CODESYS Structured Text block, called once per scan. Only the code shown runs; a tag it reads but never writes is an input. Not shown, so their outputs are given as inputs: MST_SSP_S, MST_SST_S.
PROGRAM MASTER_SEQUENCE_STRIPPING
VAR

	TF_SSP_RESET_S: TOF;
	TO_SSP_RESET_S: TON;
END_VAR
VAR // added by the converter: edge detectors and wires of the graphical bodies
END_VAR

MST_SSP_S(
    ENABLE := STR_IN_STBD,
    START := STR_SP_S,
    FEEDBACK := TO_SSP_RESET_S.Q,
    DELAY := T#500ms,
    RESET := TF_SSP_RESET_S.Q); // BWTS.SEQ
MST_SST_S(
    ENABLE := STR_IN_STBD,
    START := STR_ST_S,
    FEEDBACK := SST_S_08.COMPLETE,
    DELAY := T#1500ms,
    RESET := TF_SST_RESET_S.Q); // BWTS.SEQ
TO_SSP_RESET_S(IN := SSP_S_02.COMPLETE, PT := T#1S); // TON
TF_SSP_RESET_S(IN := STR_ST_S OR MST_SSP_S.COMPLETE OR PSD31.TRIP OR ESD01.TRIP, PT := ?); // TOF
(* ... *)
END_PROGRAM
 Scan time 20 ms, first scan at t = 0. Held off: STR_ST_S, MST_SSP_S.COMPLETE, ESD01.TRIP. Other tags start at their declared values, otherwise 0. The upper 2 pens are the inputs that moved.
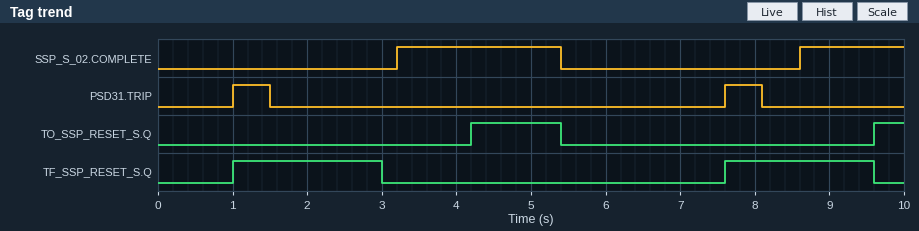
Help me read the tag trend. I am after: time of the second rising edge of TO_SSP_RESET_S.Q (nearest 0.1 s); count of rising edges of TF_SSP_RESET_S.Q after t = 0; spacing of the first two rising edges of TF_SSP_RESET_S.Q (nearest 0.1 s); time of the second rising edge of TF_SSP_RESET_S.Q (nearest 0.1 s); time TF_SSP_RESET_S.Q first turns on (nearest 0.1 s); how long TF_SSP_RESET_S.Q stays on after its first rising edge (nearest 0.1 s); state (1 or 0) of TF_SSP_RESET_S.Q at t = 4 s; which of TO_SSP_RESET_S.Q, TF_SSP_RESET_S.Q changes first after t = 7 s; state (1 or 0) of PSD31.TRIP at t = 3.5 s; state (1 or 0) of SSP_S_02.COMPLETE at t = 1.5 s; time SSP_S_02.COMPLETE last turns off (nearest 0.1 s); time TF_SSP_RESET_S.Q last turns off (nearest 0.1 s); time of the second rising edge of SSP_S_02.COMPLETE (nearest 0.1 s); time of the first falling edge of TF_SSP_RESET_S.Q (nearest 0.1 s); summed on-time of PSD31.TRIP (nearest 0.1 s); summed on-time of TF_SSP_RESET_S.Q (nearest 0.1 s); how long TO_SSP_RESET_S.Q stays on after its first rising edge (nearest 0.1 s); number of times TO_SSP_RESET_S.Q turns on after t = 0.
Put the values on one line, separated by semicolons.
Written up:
9.6 s; 2; 6.6 s; 7.6 s; 1.0 s; 2.0 s; 0; TF_SSP_RESET_S.Q; 0; 0; 5.4 s; 9.6 s; 8.6 s; 3.0 s; 1.0 s; 4.0 s; 1.2 s; 2
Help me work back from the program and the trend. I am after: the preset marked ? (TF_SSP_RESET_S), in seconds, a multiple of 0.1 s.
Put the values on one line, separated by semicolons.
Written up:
1.5 s
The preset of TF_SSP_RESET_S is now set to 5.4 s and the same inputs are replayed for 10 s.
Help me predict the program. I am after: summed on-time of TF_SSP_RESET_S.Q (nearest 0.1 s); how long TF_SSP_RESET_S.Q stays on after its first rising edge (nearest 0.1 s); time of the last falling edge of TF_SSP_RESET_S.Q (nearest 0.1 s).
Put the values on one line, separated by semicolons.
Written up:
8.3 s; 5.9 s; 6.9 s
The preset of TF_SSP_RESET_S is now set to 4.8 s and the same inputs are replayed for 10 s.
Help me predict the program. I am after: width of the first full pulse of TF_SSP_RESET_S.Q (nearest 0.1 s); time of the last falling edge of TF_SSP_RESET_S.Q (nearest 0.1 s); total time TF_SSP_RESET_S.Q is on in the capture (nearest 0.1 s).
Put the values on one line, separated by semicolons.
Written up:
5.3 s; 6.3 s; 7.7 s
